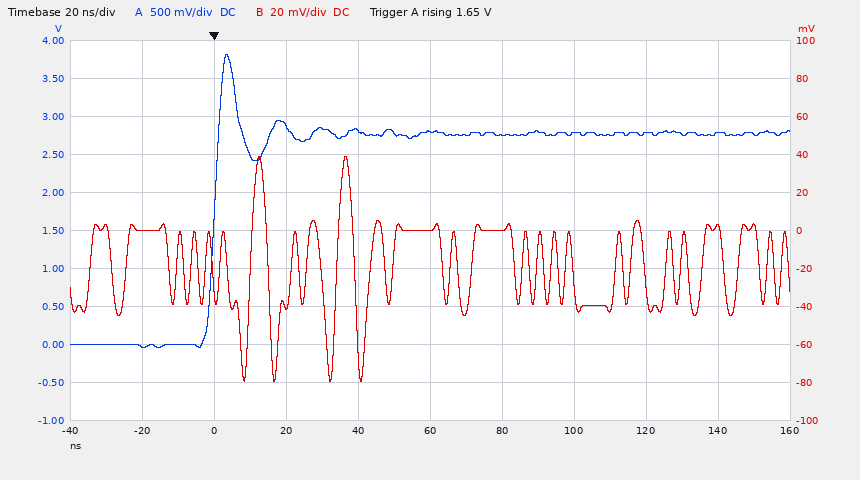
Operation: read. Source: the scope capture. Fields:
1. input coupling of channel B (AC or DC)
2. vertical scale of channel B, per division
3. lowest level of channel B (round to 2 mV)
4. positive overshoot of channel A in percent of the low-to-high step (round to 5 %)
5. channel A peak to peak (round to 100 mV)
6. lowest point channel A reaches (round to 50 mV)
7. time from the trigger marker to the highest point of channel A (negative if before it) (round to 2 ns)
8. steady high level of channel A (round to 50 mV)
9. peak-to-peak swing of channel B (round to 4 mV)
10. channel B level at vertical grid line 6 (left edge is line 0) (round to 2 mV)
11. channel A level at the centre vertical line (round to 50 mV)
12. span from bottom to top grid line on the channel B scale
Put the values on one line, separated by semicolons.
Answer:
DC; 20 mV; -80 mV; 40 %; 3.90 V; -50 mV; +4 ns; 2.75 V; 120 mV; 0 mV; 2.80 V; 200 mV
